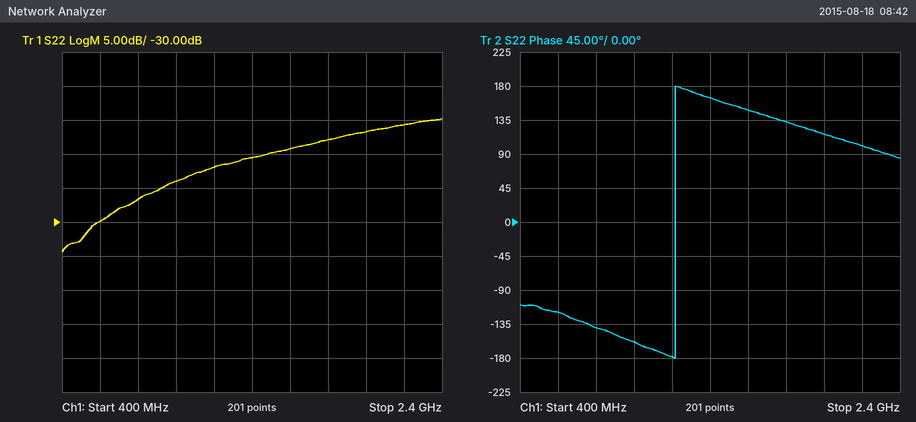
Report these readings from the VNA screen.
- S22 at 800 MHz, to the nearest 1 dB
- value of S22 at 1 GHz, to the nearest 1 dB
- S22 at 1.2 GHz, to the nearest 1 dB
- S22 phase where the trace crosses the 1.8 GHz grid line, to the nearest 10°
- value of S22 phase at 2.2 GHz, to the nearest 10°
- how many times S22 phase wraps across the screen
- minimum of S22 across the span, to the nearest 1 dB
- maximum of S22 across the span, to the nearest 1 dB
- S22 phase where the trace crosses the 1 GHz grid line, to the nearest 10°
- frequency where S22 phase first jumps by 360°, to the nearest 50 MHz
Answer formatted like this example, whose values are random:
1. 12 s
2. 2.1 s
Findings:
1. -27 dB
2. -24 dB
3. -22 dB
4. 130°
5. 100°
6. 1
7. -34 dB
8. -15 dB
9. -160°
10. 1.20 GHz
